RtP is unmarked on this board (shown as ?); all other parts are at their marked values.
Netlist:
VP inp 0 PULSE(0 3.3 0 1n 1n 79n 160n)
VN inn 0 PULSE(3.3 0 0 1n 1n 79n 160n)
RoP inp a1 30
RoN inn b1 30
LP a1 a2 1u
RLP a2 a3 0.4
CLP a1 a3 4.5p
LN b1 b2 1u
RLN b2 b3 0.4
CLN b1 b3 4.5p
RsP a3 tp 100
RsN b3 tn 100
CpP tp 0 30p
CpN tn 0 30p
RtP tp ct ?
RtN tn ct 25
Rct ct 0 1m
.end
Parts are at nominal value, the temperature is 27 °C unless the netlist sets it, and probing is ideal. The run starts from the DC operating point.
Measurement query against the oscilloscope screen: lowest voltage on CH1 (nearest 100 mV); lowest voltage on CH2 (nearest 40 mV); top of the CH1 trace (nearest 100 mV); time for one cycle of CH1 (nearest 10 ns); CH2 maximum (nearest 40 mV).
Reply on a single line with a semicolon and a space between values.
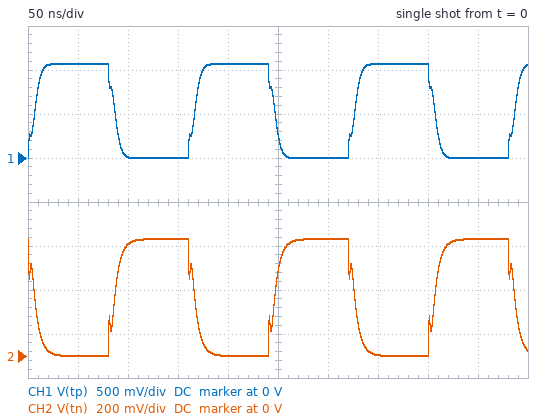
0 V; 0 V; 1.1 V; 160 ns; 520 mV
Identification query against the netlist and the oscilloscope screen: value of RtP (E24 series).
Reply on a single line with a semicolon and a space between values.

62 Ω
